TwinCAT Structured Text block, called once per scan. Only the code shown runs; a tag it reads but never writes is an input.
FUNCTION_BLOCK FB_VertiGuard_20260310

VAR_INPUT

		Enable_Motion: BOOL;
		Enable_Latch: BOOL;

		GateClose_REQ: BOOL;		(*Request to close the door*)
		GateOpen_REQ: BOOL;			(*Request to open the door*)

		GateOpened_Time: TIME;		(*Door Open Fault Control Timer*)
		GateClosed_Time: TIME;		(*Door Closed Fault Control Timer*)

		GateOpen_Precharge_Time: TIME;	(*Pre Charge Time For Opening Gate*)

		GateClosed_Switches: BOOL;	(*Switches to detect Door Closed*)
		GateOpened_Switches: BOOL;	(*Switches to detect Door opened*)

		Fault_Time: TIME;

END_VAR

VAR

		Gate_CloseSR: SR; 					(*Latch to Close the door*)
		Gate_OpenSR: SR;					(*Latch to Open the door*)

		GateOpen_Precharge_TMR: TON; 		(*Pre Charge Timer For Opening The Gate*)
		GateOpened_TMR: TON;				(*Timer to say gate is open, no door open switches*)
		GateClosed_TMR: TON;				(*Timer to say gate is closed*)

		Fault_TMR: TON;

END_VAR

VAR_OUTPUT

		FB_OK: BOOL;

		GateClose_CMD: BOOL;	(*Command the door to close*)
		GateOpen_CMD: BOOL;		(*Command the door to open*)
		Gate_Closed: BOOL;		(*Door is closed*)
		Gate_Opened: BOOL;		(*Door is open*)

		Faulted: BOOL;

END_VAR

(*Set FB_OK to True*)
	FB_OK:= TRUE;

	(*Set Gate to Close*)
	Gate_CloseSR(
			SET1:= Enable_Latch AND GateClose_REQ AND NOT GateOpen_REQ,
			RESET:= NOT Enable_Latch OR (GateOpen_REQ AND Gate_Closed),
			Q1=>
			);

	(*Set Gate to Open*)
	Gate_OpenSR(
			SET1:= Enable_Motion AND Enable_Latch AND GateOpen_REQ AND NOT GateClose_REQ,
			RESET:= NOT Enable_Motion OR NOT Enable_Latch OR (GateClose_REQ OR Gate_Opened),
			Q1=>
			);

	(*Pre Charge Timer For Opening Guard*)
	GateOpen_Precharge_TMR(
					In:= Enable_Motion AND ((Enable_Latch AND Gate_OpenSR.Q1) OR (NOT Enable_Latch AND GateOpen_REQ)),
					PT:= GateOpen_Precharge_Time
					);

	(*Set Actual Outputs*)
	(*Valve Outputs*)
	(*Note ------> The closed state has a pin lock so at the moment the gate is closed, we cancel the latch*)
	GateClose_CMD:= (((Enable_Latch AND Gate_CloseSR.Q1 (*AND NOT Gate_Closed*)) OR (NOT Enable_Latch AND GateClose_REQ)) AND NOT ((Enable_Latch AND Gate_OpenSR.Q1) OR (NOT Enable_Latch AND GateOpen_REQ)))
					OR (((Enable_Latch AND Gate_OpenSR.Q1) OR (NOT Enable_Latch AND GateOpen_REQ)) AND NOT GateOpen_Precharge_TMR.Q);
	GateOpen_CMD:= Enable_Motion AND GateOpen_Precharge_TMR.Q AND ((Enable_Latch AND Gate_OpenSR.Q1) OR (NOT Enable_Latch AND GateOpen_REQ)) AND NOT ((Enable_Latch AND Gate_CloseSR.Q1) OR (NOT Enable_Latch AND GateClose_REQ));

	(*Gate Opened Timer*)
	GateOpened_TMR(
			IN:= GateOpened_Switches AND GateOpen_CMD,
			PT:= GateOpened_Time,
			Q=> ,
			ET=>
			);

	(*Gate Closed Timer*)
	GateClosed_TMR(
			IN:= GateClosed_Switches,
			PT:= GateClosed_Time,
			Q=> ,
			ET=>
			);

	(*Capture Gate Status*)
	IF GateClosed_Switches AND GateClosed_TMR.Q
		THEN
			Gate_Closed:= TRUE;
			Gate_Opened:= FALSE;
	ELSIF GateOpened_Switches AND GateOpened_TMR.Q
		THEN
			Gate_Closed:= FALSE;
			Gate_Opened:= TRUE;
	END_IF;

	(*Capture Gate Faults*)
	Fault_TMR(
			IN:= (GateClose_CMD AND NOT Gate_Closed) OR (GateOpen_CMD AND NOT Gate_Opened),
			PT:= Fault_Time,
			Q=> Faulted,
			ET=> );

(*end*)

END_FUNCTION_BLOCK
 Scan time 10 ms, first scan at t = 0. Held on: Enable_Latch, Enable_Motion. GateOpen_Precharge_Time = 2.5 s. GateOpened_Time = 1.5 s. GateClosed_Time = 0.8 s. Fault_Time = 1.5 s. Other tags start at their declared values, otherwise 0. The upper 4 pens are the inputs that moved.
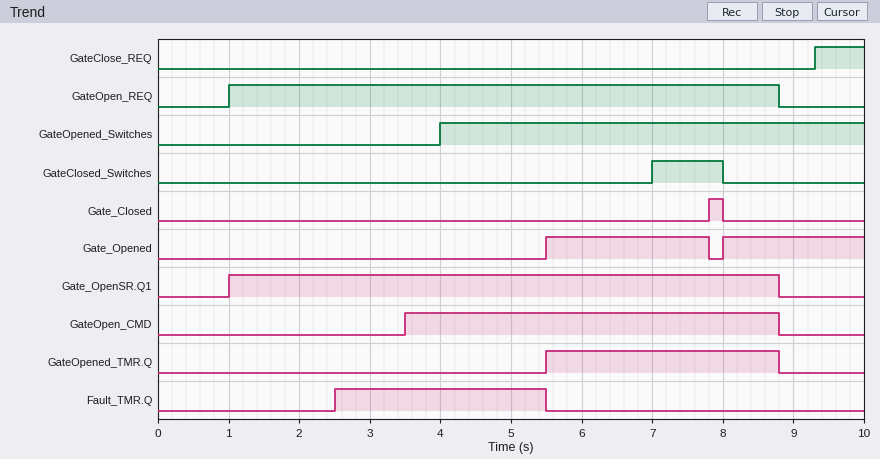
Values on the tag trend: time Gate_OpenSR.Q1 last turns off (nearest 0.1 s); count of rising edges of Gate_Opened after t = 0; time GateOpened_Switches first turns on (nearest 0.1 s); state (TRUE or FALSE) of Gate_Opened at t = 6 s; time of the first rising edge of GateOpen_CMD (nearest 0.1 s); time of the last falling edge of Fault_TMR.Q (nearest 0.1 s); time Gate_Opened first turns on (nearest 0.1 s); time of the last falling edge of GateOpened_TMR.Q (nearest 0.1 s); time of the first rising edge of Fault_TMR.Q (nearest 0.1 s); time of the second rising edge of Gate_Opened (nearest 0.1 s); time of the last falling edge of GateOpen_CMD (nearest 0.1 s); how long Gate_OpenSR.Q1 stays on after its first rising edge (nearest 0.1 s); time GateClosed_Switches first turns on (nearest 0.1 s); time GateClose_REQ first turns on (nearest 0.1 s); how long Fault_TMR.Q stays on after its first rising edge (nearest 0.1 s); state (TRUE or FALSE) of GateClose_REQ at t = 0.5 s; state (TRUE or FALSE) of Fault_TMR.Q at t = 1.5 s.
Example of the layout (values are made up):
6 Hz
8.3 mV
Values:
8.8 s
2
4.0 s
TRUE
3.5 s
5.5 s
5.5 s
8.8 s
2.5 s
8.0 s
8.8 s
7.8 s
7.0 s
9.3 s
3.0 s
FALSE
FALSE
